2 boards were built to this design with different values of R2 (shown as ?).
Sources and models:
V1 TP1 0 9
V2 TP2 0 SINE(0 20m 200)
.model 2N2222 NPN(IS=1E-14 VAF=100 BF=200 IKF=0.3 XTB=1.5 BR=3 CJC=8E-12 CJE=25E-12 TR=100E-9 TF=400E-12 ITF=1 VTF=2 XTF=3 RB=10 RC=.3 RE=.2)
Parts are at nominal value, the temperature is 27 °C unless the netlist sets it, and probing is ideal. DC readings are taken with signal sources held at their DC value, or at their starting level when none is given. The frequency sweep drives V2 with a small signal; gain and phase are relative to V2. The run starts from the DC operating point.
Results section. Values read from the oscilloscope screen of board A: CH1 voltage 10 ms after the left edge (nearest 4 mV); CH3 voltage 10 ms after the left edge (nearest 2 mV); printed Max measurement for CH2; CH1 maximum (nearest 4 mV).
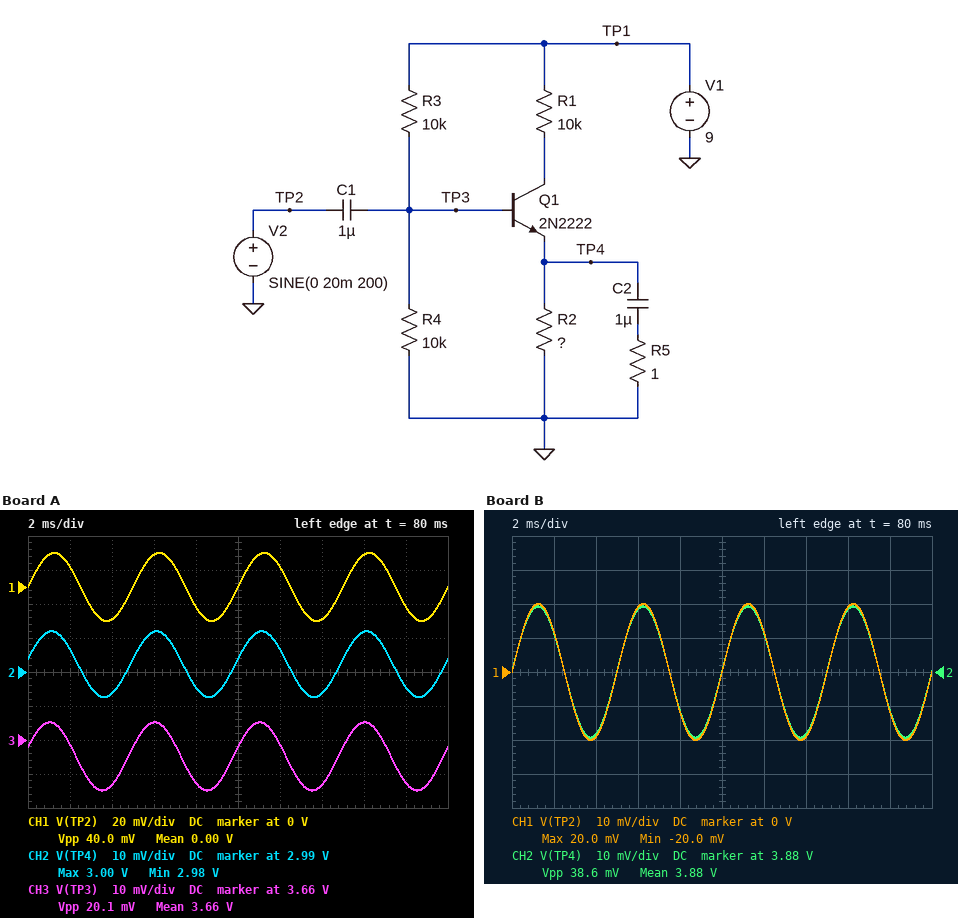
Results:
0 V
3.658 V
3.00 V
20 mV
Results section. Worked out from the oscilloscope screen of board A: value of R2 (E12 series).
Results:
3.9 kΩ
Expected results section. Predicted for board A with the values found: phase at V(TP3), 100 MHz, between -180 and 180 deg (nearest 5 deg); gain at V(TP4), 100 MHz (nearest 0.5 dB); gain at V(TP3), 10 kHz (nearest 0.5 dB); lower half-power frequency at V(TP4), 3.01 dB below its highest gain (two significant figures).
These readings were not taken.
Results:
0 deg
-28.5 dB
-0.5 dB
43 Hz
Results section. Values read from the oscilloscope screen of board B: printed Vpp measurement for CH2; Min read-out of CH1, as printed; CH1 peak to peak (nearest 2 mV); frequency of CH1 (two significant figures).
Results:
38.6 mV
-20.0 mV
40 mV
200 Hz
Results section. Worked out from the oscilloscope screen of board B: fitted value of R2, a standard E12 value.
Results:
18 kΩ
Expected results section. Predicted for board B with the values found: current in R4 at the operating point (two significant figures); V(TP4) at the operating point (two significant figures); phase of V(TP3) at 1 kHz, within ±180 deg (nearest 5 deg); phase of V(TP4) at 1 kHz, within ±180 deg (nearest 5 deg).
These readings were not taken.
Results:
450 µA
3.9 V
0 deg
-35 deg
